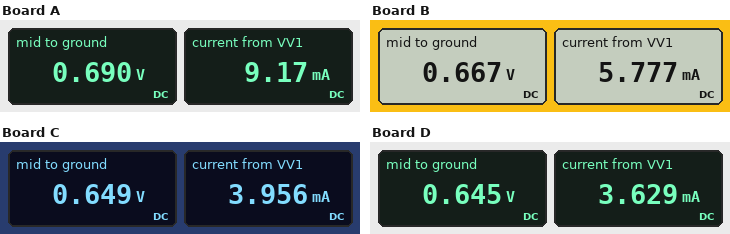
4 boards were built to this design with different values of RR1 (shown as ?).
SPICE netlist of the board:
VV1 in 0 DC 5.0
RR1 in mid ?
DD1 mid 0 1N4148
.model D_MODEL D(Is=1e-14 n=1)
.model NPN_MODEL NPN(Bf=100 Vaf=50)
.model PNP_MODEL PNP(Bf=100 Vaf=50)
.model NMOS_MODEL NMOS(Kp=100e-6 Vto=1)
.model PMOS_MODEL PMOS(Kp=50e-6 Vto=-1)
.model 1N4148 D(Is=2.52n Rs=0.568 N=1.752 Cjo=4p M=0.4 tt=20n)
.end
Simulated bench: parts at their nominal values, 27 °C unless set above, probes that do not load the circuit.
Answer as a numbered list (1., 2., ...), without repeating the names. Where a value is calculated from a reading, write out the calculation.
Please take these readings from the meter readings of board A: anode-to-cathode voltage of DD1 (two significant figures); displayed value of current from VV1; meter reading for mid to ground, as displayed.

1. 690 mV = 690 mV
2. 9.17 mA
3. 0.690 V
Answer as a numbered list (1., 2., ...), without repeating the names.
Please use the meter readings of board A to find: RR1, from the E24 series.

1. 470 Ω
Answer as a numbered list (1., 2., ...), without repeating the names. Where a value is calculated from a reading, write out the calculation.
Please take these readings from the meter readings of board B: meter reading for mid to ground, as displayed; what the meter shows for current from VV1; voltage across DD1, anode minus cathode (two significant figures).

1. 0.667 V
2. 5.777 mA
3. 667 mV = 670 mV
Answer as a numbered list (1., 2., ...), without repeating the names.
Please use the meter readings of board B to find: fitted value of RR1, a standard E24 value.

1. 750 Ω
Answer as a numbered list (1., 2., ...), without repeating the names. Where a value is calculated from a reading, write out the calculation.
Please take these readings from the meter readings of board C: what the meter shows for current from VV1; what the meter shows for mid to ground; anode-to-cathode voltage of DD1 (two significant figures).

1. 3.956 mA
2. 0.649 V
3. 649 mV = 650 mV
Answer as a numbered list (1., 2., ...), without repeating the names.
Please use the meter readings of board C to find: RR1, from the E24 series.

1. 1.1 kΩ
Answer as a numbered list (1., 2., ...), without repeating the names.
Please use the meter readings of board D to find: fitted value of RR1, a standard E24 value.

1. 1.2 kΩ
